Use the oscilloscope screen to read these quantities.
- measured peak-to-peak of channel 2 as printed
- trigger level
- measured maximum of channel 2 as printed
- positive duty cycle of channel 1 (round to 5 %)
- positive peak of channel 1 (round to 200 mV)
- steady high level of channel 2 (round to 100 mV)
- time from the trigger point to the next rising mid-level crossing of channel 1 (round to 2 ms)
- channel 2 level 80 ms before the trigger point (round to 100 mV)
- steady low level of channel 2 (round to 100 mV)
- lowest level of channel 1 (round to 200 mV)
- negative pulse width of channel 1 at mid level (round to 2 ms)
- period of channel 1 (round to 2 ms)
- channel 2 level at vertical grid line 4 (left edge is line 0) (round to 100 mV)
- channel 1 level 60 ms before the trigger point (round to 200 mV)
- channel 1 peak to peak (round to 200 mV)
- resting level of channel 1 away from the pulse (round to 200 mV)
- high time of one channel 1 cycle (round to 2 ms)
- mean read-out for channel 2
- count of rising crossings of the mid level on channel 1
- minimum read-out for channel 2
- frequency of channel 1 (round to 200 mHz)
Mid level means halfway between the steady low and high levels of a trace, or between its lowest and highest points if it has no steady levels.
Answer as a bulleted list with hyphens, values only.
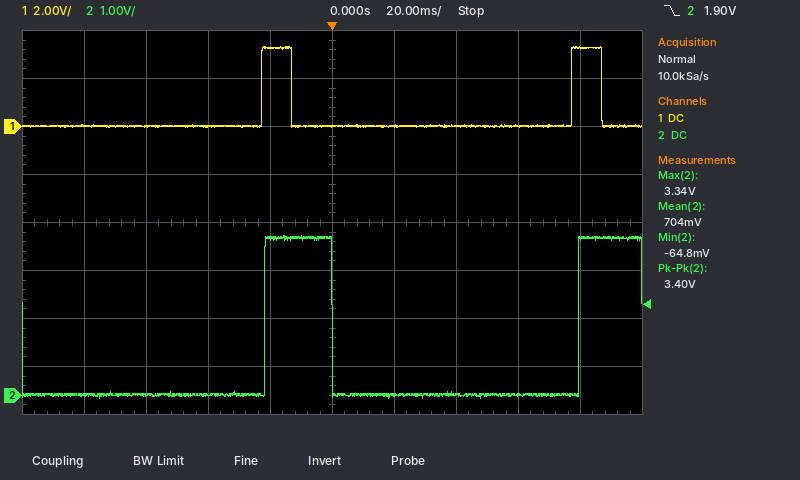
- 3.40 V
- 1.90 V
- 3.34 V
- 10 %
- 3.4 V
- 3.3 V
- 78 ms
- 0.0 V
- 0.0 V
- 0.0 V
- 90 ms
- 100 ms
- 3.3 V
- 0.0 V
- 3.4 V
- 0.0 V
- 10 ms
- 704 mV
- 2
- -64.8 mV
- 10.0 Hz
